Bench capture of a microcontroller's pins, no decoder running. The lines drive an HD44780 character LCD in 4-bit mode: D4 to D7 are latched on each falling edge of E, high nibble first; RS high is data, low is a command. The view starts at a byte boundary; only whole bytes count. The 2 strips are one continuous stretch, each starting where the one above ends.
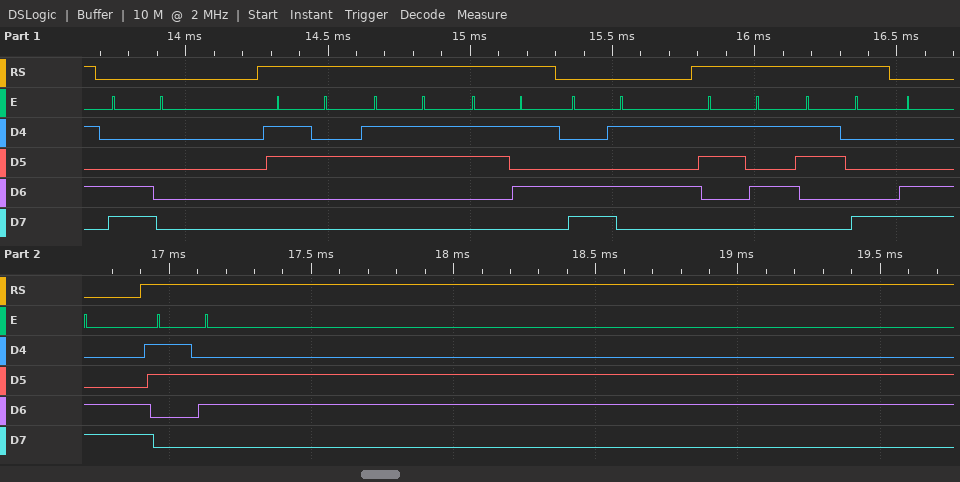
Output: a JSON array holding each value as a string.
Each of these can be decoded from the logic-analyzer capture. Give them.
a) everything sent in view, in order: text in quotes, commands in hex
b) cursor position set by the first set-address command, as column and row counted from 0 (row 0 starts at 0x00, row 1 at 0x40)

["0xC0 \"235\" 0xC5 \"58\" 0xCC \"6\"", "column 0, row 1"]
